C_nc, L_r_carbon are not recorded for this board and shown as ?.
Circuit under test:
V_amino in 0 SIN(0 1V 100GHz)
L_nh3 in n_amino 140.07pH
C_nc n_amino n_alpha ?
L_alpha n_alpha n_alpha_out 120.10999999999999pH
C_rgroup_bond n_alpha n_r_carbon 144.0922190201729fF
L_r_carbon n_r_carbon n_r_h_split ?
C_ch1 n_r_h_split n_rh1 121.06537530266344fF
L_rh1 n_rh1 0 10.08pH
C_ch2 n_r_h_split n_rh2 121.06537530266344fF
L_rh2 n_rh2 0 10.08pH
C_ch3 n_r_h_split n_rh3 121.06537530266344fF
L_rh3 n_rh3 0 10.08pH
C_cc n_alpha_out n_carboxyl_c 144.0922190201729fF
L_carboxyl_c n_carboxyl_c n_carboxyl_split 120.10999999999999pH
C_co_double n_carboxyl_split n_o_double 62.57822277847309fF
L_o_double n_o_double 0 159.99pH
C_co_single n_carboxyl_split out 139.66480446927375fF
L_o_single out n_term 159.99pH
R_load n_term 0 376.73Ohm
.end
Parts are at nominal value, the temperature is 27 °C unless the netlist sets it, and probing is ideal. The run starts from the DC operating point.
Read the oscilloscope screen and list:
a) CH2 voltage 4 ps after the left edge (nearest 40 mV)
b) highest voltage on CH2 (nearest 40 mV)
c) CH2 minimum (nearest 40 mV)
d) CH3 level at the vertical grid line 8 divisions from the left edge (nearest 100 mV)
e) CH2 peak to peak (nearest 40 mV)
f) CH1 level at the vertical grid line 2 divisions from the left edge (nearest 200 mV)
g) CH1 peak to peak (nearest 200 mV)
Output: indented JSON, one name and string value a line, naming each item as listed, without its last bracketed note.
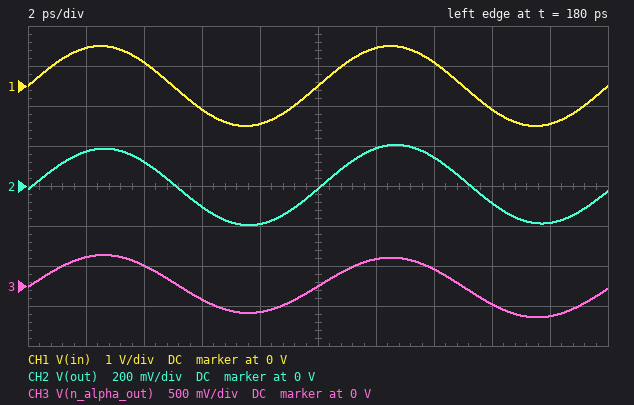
{
  "CH2 voltage 4 ps after the left edge": "120 mV",
  "highest voltage on CH2": "200 mV",
  "CH2 minimum": "-200 mV",
  "CH3 level at the vertical grid line 8 divisions from the left edge": "-200 mV",
  "CH2 peak to peak": "400 mV",
  "CH1 level at the vertical grid line 2 divisions from the left edge": "600 mV",
  "CH1 peak to peak": "2.0 V"
}
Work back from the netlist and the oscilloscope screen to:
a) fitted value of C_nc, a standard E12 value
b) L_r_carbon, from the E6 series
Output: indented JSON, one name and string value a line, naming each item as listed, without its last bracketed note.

{
  "fitted value of C_nc, a standard E12 value": "56 fF",
  "L_r_carbon, from the E6 series": "220 pH"
}
